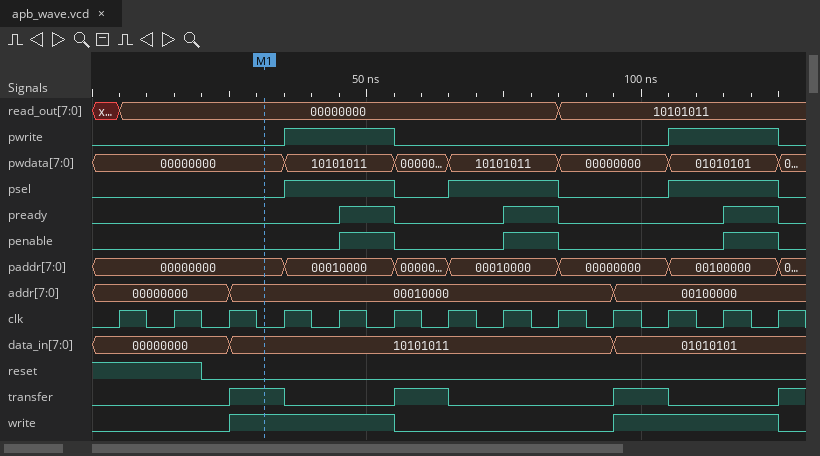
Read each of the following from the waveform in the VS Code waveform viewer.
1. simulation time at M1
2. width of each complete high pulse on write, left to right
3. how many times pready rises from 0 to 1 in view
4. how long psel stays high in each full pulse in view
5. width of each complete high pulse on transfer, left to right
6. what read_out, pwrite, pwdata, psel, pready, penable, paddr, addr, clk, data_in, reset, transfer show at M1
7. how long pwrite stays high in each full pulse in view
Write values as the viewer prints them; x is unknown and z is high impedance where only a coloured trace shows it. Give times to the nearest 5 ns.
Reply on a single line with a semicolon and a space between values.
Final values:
30 ns; 30 ns, 30 ns; 3; 20 ns, 20 ns, 20 ns; 10 ns, 10 ns, 10 ns; read_out=00000000, pwrite=0, pwdata=00000000, psel=0, pready=0, penable=0, paddr=00000000, addr=00010000, clk=0, data_in=10101011, reset=0, transfer=1; 20 ns, 20 ns
